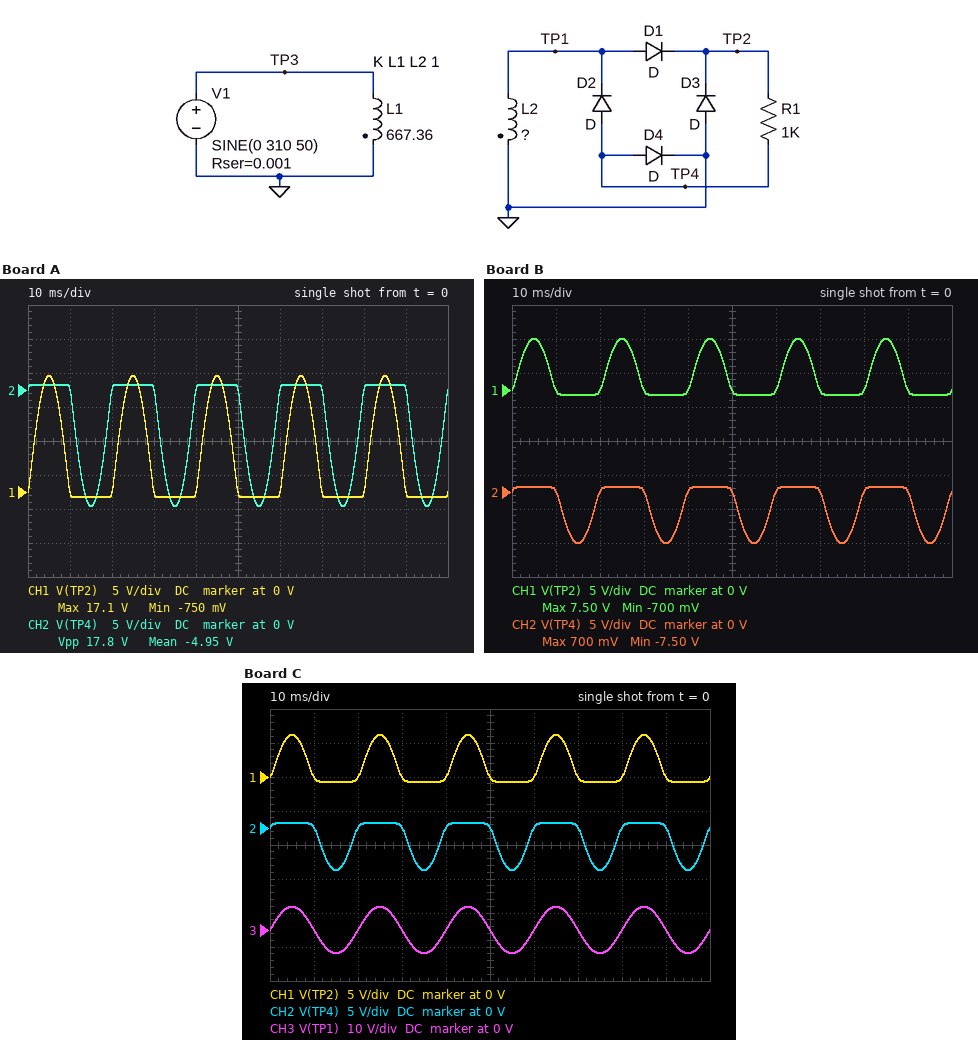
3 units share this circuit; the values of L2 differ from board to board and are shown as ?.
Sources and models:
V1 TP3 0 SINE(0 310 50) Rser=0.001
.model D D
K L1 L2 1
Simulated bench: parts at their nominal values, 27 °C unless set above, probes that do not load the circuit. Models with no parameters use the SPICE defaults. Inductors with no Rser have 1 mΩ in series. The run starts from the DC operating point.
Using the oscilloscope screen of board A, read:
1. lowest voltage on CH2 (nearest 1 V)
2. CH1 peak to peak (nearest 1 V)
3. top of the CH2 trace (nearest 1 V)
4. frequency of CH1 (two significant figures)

-17 V
18 V
1 V
50 Hz
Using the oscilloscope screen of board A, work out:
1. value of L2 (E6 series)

2.2 H
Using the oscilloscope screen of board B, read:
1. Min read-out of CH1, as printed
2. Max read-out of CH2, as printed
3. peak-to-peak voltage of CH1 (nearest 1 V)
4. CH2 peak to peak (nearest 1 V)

-700 mV
700 mV
8 V
8 V
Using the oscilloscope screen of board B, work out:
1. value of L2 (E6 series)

470 mH
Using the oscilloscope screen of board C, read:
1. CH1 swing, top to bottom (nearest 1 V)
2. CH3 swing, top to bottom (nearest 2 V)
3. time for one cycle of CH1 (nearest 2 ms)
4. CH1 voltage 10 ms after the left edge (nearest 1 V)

7 V
14 V
20 ms
0 V
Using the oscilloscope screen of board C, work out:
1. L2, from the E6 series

330 mH
